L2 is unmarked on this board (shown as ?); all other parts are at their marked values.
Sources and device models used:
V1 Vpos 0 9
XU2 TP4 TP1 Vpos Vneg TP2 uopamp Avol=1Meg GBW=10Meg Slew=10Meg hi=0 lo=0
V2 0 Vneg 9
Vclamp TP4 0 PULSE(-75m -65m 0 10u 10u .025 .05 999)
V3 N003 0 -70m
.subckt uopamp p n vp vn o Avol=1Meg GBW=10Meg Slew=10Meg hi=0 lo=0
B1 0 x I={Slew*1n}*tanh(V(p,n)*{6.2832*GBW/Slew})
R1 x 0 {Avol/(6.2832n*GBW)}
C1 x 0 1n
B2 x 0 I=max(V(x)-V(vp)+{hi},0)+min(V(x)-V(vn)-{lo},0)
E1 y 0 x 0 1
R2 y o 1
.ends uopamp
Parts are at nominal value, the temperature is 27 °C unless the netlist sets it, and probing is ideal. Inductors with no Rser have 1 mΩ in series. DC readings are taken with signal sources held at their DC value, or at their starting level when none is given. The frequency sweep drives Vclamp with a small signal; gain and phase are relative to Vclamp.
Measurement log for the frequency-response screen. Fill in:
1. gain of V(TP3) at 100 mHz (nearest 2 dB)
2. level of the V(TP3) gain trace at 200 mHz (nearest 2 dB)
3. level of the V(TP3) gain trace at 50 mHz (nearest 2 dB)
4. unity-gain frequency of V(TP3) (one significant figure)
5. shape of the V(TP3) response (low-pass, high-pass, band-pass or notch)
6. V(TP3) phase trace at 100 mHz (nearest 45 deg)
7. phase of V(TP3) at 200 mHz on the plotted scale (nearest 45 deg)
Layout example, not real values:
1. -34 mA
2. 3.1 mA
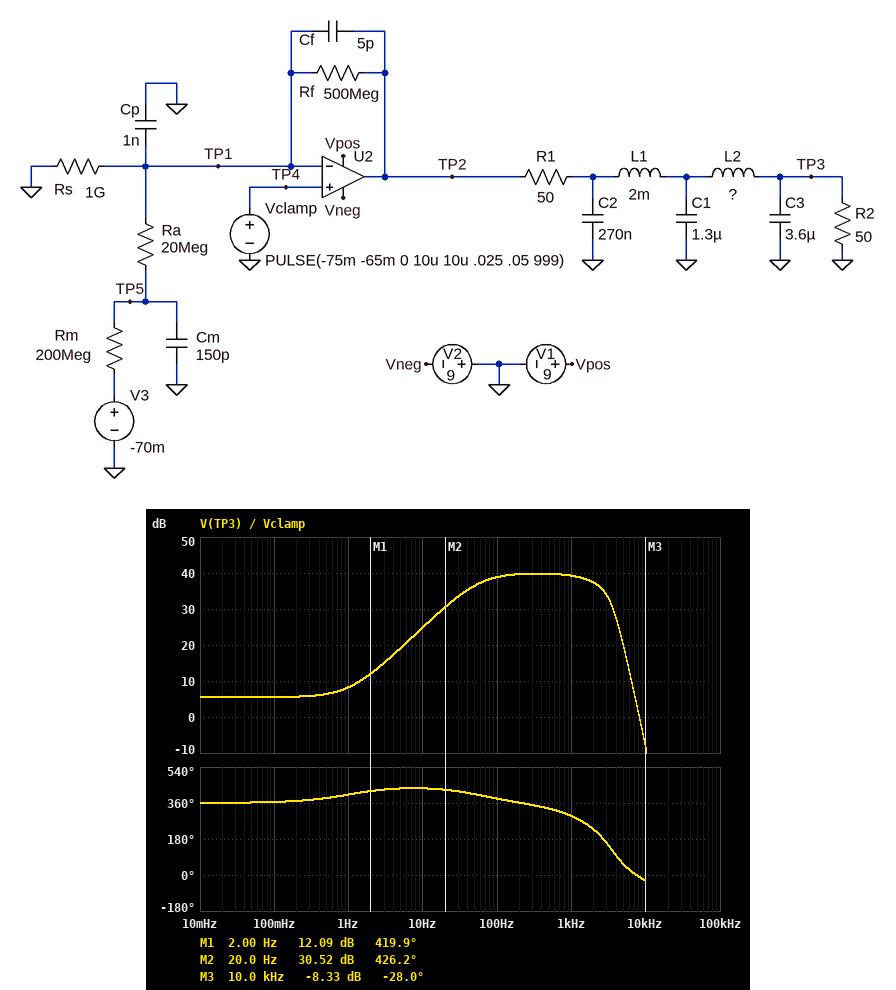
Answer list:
1. 6 dB
2. 6 dB
3. 6 dB
4. 8 kHz
5. band-pass
6. 360 deg
7. 360 deg
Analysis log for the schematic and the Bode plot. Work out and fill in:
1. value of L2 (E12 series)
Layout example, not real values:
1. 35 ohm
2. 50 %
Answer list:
1. 3.9 mH
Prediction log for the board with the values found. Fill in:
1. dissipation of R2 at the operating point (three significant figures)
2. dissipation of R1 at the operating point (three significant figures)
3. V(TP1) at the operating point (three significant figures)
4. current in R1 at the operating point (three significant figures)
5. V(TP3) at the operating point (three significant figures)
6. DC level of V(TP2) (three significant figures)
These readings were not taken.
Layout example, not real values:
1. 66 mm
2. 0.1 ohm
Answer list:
1. 76.7 µW
2. 76.7 µW
3. -75.0 mV
4. 1.24 mA
5. -61.9 mV
6. -124 mV
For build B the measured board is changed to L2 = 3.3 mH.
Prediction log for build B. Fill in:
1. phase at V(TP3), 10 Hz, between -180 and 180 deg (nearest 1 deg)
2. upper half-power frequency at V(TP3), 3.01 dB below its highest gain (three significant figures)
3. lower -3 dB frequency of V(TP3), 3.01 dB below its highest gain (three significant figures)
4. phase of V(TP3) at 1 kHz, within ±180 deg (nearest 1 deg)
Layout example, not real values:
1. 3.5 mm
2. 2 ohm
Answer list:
1. 73 deg
2. 2.30 kHz
3. 53.6 Hz
4. -62 deg
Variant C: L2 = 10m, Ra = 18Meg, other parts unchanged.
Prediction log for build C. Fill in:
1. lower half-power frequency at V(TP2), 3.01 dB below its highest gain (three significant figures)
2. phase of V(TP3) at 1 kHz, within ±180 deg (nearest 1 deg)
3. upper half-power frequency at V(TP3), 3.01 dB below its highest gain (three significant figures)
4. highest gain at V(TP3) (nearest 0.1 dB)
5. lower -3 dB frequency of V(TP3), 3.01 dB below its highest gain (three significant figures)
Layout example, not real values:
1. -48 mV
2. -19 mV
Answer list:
1. 55.5 Hz
2. -95 deg
3. 1.33 kHz
4. 39.9 dB
5. 54.2 Hz
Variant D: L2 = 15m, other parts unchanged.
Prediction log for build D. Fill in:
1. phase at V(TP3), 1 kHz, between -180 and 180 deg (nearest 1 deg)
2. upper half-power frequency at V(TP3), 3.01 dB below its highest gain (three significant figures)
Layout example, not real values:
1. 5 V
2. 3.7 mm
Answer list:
1. -114 deg
2. 1.04 kHz
